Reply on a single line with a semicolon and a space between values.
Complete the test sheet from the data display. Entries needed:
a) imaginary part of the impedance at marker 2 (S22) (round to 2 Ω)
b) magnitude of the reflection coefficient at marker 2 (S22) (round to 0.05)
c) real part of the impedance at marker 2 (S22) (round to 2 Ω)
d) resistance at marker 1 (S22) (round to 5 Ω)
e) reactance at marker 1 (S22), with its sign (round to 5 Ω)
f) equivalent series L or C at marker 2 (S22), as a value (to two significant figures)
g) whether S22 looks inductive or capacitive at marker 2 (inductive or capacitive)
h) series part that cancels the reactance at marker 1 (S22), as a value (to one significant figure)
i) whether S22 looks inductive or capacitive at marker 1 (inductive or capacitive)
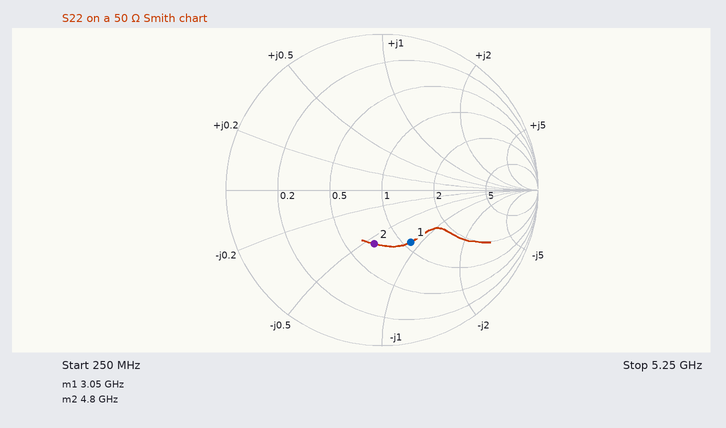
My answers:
-28 Ω; 0.35; 36 Ω; 55 Ω; -45 Ω; 1.2 pF; capacitive; 2 nH; capacitive
